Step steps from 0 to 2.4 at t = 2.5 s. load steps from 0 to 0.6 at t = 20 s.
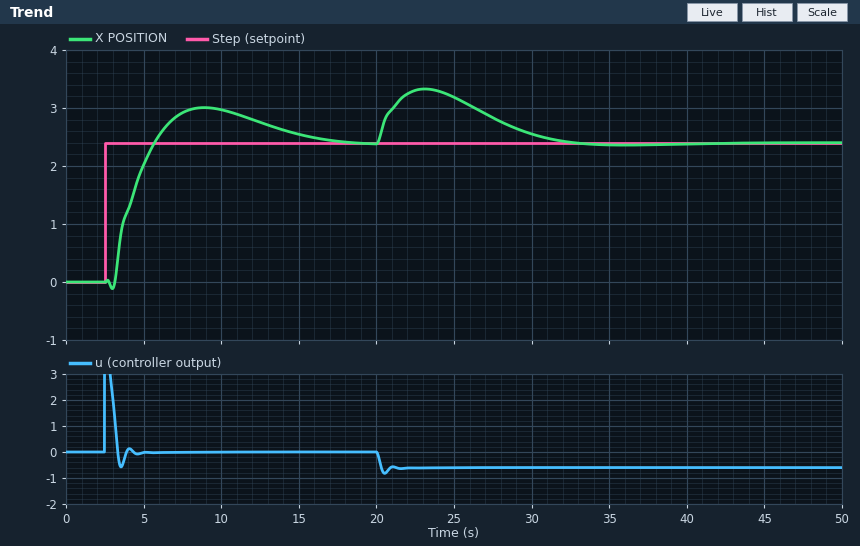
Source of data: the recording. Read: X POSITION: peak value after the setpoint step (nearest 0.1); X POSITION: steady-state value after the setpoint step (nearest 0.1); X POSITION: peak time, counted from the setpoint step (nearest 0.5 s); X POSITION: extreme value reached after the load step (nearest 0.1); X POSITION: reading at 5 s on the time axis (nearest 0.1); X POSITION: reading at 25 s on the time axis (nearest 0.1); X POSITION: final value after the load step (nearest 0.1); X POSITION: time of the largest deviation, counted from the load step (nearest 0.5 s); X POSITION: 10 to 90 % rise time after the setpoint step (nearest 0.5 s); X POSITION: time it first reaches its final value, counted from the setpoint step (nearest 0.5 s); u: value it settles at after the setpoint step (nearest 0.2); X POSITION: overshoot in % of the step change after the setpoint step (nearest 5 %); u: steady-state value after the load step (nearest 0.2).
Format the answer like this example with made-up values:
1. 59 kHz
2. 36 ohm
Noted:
1. 3.0
2. 2.4
3. 6.5 s
4. 3.3
5. 2.0
6. 3.2
7. 2.4
8. 3.0 s
9. 2.0 s
10. 3.0 s
11. 0.0
12. 25 %
13. -0.6
